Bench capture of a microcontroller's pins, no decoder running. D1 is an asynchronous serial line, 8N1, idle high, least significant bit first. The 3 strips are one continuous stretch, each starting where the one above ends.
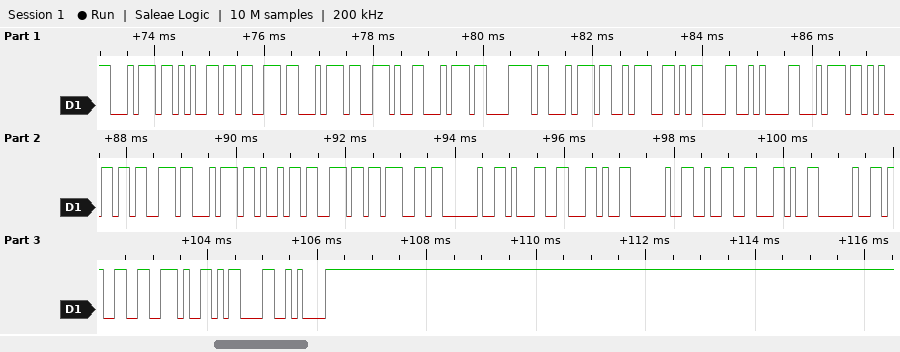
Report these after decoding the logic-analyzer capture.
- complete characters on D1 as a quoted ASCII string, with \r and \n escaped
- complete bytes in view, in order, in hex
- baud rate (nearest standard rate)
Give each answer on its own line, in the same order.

"test.txt:\r\ntesting 1, 2, 3.\r\n"
0x74 0x65 0x73 0x74 0x2E 0x74 0x78 0x74 0x3A 0x0D 0x0A 0x74 0x65 0x73 0x74 0x69 0x6E 0x67 0x20 0x31 0x2C 0x20 0x32 0x2C 0x20 0x33 0x2E 0x0D 0x0A
9600 baud
